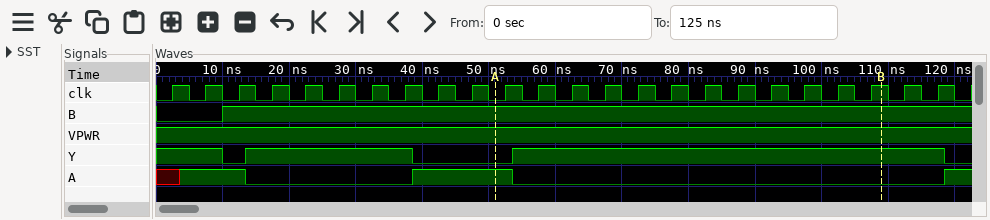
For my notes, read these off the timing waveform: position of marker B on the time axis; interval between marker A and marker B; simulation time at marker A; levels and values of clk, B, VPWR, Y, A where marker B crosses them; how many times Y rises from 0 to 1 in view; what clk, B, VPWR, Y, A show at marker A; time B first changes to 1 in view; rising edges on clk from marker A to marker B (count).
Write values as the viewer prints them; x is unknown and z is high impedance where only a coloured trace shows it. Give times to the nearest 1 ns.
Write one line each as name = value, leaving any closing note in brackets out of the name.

position of marker B on the time axis = 109 ns
interval between marker A and marker B = 58 ns
simulation time at marker A = 51 ns
levels and values of clk, B, VPWR, Y, A where marker B crosses them = clk=1, B=1, VPWR=1, Y=1, A=0
how many times Y rises from 0 to 1 in view = 2
what clk, B, VPWR, Y, A show at marker A = clk=0, B=1, VPWR=1, Y=0, A=1
time B first changes to 1 in view = 10 ns
rising edges on clk from marker A to marker B = 12
